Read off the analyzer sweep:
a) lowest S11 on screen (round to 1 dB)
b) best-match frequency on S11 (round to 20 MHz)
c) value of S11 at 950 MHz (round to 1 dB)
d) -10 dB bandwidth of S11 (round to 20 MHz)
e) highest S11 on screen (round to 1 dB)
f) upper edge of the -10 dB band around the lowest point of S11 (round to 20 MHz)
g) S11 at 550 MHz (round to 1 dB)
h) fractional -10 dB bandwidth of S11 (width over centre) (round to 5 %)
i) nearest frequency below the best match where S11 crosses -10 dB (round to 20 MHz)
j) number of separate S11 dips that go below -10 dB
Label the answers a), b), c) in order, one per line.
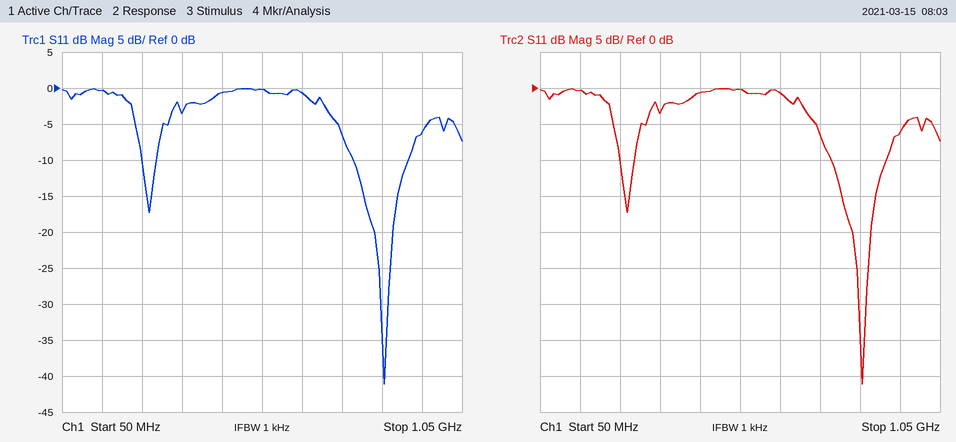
a) -41 dB
b) 860 MHz
c) -6 dB
d) 140 MHz
e) 0 dB
f) 920 MHz
g) 0 dB
h) 15 %
i) 780 MHz
j) 2
